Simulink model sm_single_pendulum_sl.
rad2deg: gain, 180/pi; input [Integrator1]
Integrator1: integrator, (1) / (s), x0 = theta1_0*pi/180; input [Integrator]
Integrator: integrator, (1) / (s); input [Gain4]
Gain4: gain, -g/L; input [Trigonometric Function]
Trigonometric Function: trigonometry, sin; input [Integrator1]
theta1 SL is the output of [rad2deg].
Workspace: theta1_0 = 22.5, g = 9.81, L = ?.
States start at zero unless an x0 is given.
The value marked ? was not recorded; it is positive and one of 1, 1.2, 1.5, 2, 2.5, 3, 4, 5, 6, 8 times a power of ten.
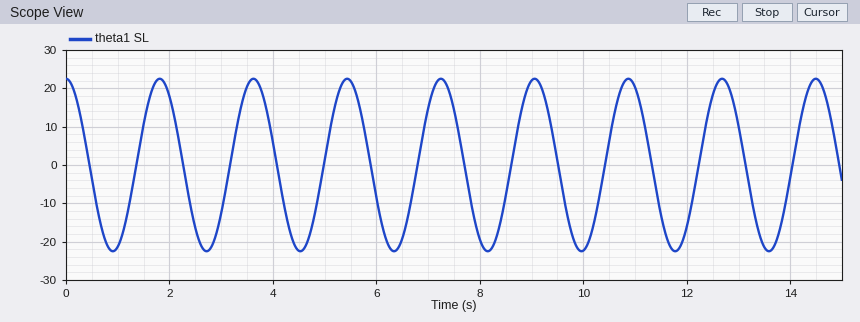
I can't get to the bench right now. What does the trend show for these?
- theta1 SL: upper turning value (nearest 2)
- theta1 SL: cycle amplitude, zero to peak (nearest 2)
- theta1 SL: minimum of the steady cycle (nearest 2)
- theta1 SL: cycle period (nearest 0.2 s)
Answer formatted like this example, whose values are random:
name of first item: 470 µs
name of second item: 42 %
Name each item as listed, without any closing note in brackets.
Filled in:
theta1 SL: upper turning value: 22
theta1 SL: cycle amplitude, zero to peak: 22
theta1 SL: minimum of the steady cycle: -22
theta1 SL: cycle period: 1.8 s
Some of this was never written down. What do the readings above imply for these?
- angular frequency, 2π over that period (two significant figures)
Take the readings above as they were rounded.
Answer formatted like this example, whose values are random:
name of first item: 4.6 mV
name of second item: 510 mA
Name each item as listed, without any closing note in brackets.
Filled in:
angular frequency, 2π over that period: 3.5 rad/s
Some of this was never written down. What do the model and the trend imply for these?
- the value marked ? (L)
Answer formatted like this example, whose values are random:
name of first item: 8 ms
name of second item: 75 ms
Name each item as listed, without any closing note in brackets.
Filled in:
the value marked ?: 0.8
